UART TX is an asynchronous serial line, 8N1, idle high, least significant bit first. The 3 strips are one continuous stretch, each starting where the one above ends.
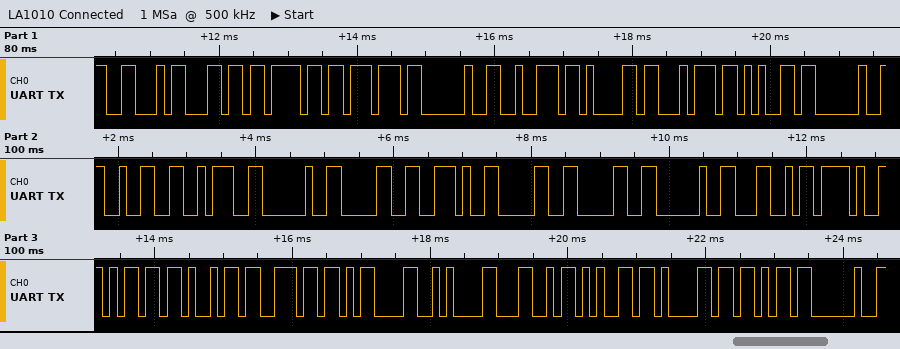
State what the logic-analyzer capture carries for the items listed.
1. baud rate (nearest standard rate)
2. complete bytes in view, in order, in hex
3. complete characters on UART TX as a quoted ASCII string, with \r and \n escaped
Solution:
9600 baud
0x46 0x6C 0x6F 0x77 0x20 0x72 0x61 0x74 0x65 0x20 0x32 0x3A 0x20 0x30 0x2E 0x30 0x30 0x20 0x4C 0x2F 0x6D 0x69 0x6E 0x0D 0x0A 0x4C 0x65 0x61 0x6B 0x20
"Flow rate 2: 0.00 L/min\r\nLeak "
